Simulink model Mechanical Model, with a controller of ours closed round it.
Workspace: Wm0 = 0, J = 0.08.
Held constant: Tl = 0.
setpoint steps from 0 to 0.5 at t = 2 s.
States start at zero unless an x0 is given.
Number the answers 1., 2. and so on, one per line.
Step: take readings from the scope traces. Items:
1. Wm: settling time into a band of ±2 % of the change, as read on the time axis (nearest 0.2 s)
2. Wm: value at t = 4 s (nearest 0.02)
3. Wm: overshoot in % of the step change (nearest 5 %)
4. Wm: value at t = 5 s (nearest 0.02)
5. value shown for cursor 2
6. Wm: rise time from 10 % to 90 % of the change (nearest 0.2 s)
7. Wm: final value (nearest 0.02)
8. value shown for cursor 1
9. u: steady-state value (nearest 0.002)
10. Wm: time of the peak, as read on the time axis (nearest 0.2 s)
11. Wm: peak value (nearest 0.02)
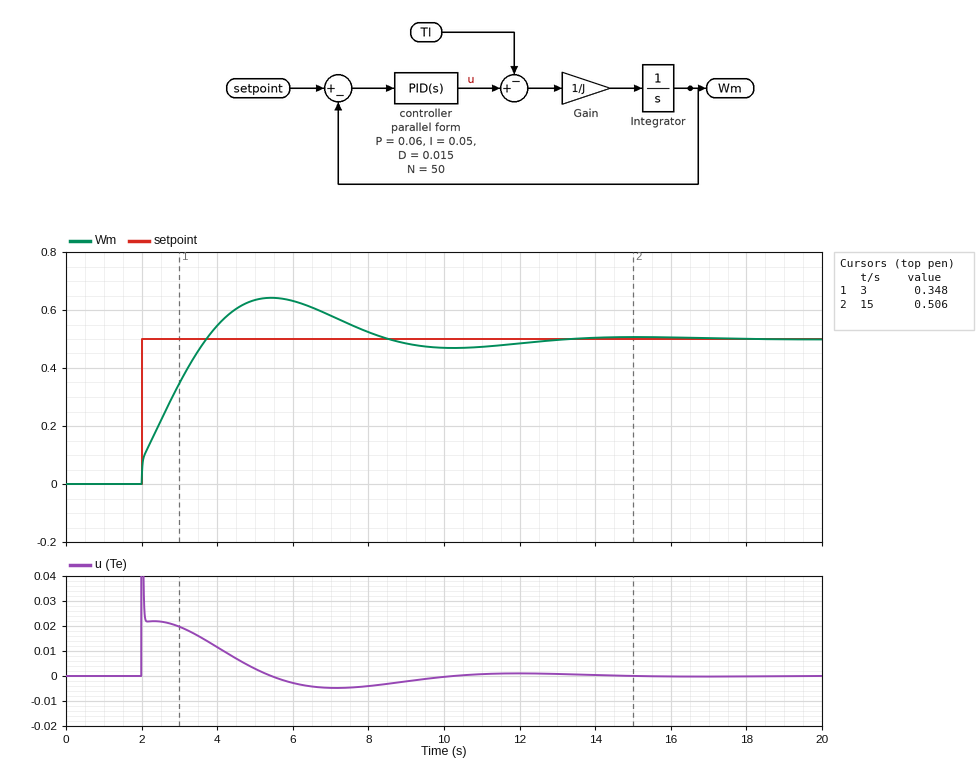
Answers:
1. 12.4 s
2. 0.54
3. 30 %
4. 0.64
5. 0.506
6. 1.4 s
7. 0.50
8. 0.348
9. 0.000
10. 5.4 s
11. 0.64
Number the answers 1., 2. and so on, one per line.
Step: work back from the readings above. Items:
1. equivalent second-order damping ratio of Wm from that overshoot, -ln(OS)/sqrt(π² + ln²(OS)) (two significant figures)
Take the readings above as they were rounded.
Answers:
1. 0.36
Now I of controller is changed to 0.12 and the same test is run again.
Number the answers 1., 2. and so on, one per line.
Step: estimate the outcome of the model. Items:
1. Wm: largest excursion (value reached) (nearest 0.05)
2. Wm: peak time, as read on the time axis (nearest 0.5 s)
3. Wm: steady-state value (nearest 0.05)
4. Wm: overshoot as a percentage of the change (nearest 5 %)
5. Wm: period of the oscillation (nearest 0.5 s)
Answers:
1. 0.70
2. 4.5 s
3. 0.50
4. 40 %
5. 6.0 s
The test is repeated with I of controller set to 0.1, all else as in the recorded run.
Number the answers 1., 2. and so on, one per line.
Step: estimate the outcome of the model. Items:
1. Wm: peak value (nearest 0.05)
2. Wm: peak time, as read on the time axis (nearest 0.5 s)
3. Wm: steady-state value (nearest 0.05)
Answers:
1. 0.70
2. 4.5 s
3. 0.50
